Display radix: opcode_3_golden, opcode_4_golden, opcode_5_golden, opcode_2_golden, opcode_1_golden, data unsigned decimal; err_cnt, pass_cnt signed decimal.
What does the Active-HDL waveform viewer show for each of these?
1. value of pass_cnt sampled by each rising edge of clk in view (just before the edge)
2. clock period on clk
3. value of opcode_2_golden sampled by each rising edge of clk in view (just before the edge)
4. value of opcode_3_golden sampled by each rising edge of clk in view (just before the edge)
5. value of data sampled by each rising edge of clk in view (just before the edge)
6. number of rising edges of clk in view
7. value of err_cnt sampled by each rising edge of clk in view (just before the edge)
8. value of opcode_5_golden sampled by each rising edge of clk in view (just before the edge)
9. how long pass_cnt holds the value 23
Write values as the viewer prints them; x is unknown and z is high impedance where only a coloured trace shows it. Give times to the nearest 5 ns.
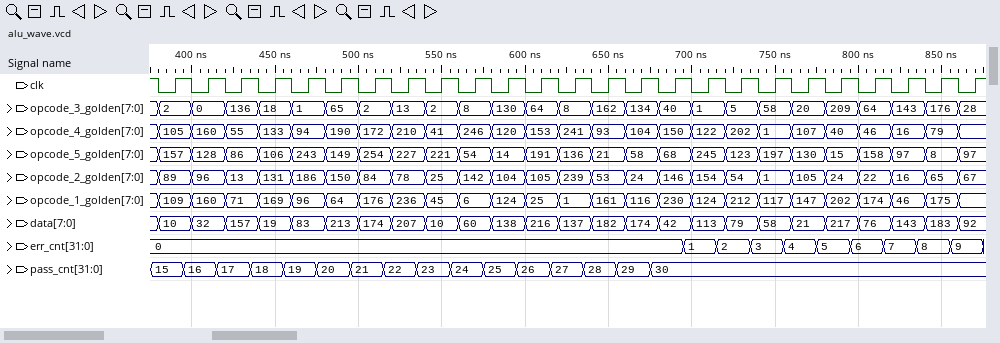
15, 16, 17, 18, 19, 20, 21, 22, 23, 24, 25, 26, 27, 28, 29, 30, 30, 30, 30, 30, 30, 30, 30, 30, 30
20 ns
89, 96, 13, 131, 186, 150, 84, 78, 25, 142, 104, 105, 239, 53, 24, 146, 154, 54, 1, 105, 24, 22, 16, 65, 67
2, 0, 136, 18, 1, 65, 2, 13, 2, 8, 130, 64, 8, 162, 134, 40, 1, 5, 58, 20, 209, 64, 143, 176, 28
10, 32, 157, 19, 83, 213, 174, 207, 10, 60, 138, 216, 137, 182, 174, 42, 113, 79, 58, 21, 217, 76, 143, 183, 92
25
0, 0, 0, 0, 0, 0, 0, 0, 0, 0, 0, 0, 0, 0, 0, 0, 1, 2, 3, 4, 5, 6, 7, 8, 9
157, 128, 86, 106, 243, 149, 254, 227, 221, 54, 14, 191, 136, 21, 58, 68, 245, 123, 197, 130, 15, 158, 97, 8, 97
20 ns
